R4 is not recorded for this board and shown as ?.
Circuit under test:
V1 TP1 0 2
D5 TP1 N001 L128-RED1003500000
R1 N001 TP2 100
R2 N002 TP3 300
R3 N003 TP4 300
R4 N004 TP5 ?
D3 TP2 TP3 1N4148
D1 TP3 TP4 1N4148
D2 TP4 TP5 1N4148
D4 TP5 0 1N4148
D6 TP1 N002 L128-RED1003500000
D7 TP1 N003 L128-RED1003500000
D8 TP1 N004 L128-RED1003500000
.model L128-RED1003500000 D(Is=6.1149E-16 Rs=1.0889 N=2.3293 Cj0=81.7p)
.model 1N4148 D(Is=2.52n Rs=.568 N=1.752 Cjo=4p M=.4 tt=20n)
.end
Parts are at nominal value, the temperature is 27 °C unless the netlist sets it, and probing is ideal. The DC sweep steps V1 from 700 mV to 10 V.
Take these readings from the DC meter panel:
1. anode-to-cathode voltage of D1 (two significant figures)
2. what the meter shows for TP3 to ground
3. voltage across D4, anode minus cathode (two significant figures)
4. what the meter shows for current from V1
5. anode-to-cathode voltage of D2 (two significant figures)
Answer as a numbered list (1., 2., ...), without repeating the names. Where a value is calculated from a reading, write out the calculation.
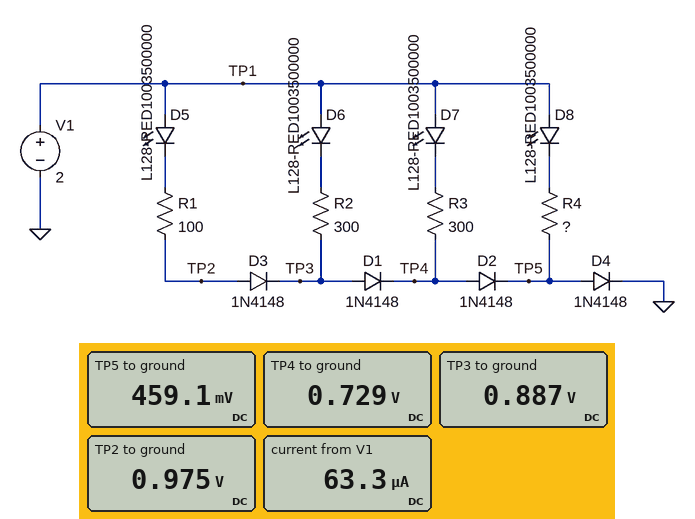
1. 887 mV - 729 mV = 160 mV
2. 0.887 V
3. 459.1 mV = 460 mV
4. 63.3 µA
5. 729 mV - 459.1 mV = 270 mV
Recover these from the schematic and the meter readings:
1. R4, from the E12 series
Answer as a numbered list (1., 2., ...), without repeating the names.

1. 220 Ω
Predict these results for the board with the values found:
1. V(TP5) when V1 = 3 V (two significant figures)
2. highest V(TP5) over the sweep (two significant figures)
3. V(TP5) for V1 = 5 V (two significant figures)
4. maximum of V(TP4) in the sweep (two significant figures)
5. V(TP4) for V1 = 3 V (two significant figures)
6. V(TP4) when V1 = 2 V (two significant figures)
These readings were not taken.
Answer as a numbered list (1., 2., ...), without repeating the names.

1. 640 mV
2. 870 mV
3. 740 mV
4. 1.7 V
5. 1.2 V
6. 730 mV
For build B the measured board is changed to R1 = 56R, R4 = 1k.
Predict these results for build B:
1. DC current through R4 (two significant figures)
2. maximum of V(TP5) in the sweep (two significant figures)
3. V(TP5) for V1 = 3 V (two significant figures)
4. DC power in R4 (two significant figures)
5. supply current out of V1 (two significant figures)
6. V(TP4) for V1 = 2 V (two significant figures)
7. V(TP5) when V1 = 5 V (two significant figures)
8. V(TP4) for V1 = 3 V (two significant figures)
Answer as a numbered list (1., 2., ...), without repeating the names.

1. 46 µA
2. 880 mV
3. 600 mV
4. 2.1 µW
5. 47 µA
6. 720 mV
7. 730 mV
8. 1.2 V
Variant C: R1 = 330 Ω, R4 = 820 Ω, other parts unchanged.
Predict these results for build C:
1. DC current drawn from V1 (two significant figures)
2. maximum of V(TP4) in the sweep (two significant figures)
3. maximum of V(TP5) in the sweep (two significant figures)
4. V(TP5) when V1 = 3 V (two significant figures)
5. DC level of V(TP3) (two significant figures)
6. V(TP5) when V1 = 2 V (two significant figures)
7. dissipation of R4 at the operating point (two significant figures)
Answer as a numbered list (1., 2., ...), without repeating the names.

1. 50 µA
2. 1.6 V
3. 810 mV
4. 600 mV
5. 880 mV
6. 450 mV
7. 1.9 µW
